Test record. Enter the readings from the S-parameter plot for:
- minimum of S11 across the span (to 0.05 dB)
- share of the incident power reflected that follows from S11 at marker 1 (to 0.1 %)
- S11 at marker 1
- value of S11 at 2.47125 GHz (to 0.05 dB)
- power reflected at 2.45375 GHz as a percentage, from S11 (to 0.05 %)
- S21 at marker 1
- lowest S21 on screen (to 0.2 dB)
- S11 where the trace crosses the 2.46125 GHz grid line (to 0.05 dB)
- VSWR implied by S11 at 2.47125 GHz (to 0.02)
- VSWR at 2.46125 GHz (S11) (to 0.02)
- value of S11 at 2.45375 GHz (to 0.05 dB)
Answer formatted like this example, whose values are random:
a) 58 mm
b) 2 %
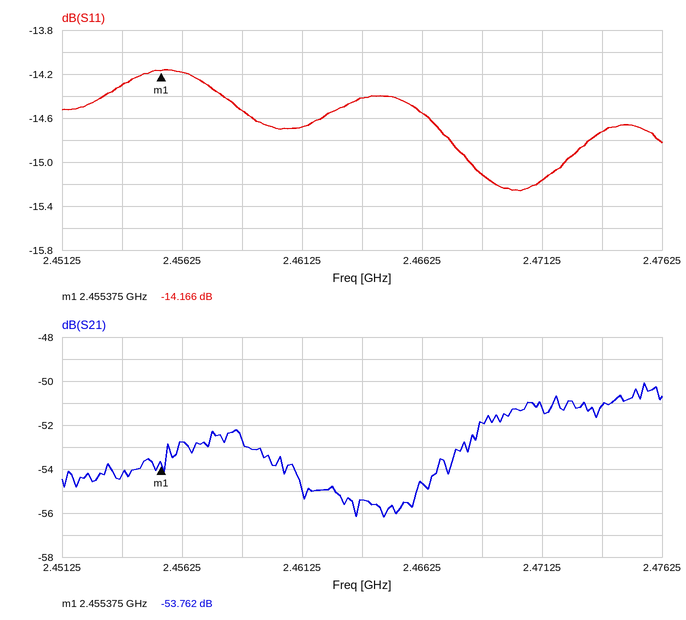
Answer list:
a) -15.25 dB
b) 3.8 %
c) -14.166 dB
d) -15.15 dB
e) 3.70 %
f) -53.762 dB
g) -56.2 dB
h) -14.70 dB
i) 1.42
j) 1.46
k) -14.30 dB
